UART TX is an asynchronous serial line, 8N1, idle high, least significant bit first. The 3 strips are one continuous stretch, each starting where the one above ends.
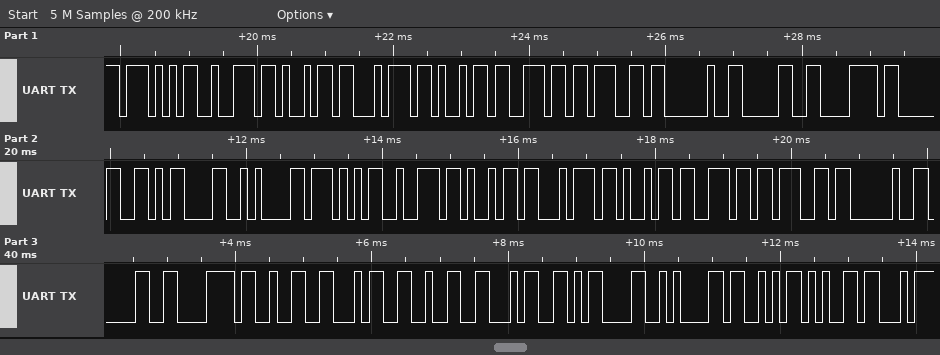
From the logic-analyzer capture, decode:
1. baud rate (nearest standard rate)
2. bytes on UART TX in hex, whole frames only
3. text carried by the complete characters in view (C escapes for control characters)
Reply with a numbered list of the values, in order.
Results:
1. 9600 baud
2. 57 72 69 74 69 6E 67 20 30 78 30 0D 0A 57 72 69 74 69 6E 67 20 30 78 32 34 32 34 0D 0A 53 65
3. "Writing 0x0\r\nWriting 0x2424\r\nSe"
